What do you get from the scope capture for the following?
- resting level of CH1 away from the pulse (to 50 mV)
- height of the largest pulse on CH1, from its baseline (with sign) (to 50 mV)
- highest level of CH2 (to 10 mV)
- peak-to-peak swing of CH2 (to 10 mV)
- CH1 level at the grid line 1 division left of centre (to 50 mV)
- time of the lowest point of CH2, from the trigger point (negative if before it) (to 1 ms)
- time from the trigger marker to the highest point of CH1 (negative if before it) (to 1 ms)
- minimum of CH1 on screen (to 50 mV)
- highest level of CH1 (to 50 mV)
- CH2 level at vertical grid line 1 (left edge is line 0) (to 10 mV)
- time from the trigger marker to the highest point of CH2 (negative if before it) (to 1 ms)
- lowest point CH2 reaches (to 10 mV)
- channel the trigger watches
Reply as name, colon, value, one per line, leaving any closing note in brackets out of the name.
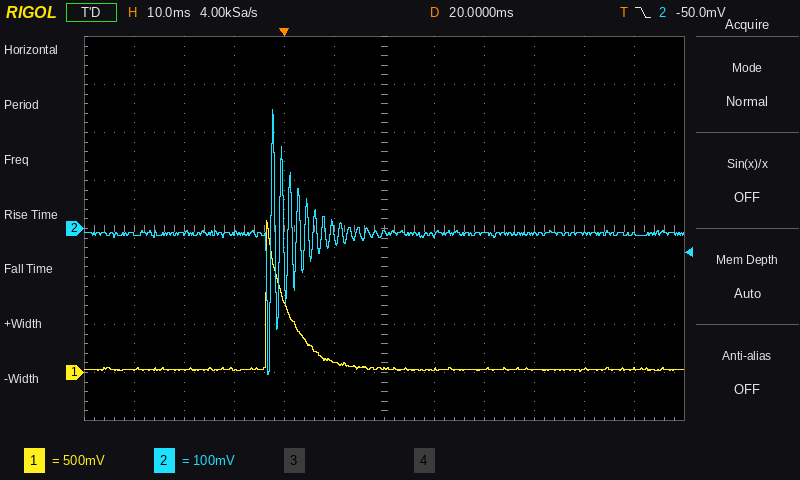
resting level of CH1 away from the pulse: 50 mV
height of the largest pulse on CH1, from its baseline (with sign): +1.55 V
highest level of CH2: 250 mV
peak-to-peak swing of CH2: 550 mV
CH1 level at the grid line 1 division left of centre: 100 mV
time of the lowest point of CH2, from the trigger point (negative if before it): -3 ms
time from the trigger marker to the highest point of CH1 (negative if before it): -3 ms
minimum of CH1 on screen: 0 mV
highest level of CH1: 1.60 V
CH2 level at vertical grid line 1 (left edge is line 0): -10 mV
time from the trigger marker to the highest point of CH2 (negative if before it): -2 ms
lowest point CH2 reaches: -300 mV
channel the trigger watches: CH2
